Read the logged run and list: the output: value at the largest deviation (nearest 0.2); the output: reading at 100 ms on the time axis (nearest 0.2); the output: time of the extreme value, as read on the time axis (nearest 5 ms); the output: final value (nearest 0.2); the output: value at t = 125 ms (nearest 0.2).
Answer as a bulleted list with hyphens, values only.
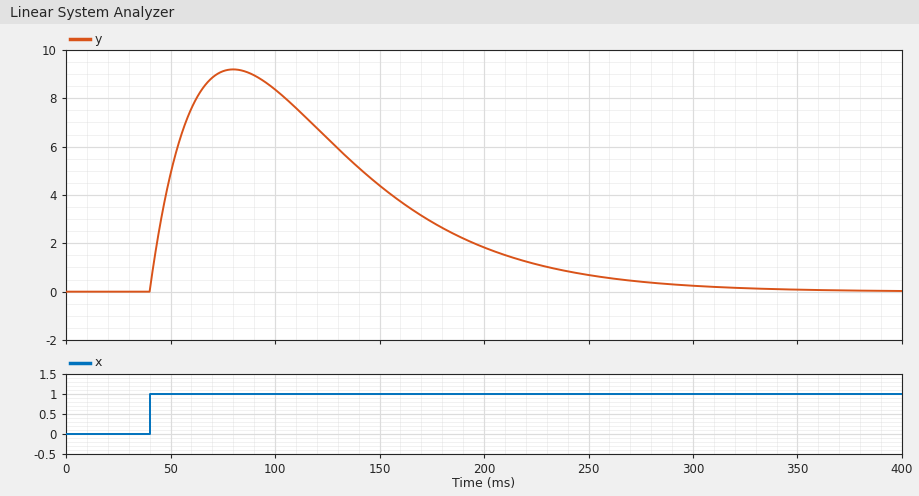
- 9.2
- 8.4
- 80 ms
- 0.0
- 6.4
